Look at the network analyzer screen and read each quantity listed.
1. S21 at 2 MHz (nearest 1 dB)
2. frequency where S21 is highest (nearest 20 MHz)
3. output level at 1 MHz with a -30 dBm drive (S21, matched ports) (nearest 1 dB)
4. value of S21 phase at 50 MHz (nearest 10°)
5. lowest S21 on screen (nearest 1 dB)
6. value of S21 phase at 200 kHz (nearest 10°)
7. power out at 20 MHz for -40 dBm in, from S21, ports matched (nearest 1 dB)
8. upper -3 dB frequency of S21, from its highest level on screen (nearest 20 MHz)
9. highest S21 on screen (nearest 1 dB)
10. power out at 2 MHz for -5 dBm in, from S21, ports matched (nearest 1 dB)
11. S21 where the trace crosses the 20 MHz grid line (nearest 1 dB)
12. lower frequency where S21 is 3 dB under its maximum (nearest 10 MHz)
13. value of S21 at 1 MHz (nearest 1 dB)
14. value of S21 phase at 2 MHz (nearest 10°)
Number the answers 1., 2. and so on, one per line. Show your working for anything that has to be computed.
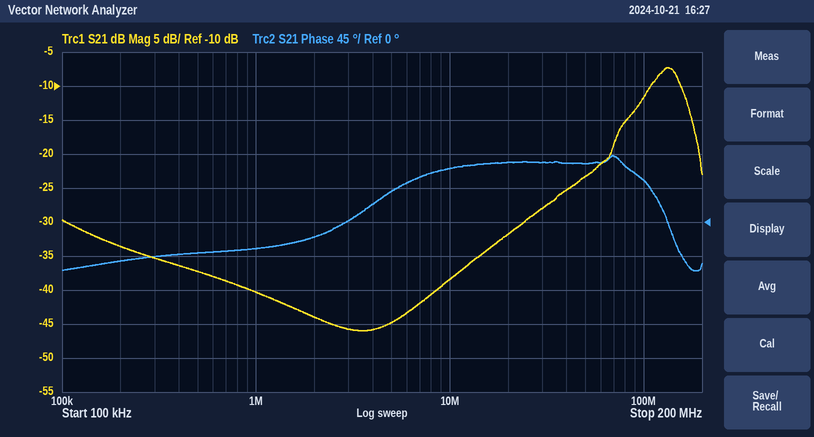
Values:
1. -44 dB
2. 140 MHz
3. -30 dBm + (-40 dB) = -70 dBm
4. 80°
5. -46 dB
6. -50°
7. -40 dBm + (-32 dB) = -72 dBm
8. 160 MHz
9. -7 dB
10. -5 dBm + (-44 dB) = -49 dBm
11. -32 dB
12. 110 MHz
13. -40 dB
14. -20°
